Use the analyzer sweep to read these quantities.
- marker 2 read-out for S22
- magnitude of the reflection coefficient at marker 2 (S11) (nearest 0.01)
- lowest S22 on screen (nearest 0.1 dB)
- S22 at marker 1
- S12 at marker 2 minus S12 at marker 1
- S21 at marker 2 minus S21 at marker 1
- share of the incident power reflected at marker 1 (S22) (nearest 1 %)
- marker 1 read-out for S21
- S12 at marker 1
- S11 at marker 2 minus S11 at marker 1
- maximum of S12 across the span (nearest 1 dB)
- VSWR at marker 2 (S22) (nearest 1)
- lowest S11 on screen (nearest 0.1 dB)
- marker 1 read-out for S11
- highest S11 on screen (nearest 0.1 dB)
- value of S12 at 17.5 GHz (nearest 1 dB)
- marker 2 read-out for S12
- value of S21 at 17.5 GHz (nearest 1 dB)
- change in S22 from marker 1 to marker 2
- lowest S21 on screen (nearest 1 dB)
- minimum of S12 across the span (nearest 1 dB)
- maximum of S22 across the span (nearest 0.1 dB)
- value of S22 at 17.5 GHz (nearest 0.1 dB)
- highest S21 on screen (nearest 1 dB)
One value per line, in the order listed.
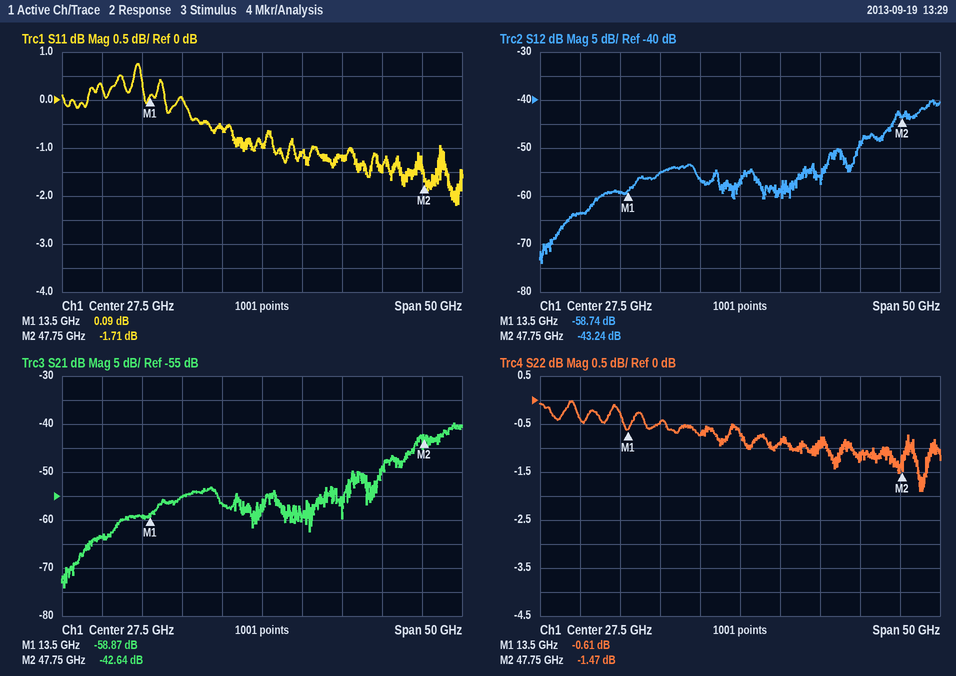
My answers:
-1.47 dB
0.82
-1.9 dB
-0.61 dB
15.50 dB
16.23 dB
87 %
-58.87 dB
-58.74 dB
-1.80 dB
-40 dB
12
-2.2 dB
0.09 dB
0.8 dB
-55 dB
-43.24 dB
-55 dB
-0.86 dB
-74 dB
-74 dB
0.0 dB
-0.5 dB
-40 dB
